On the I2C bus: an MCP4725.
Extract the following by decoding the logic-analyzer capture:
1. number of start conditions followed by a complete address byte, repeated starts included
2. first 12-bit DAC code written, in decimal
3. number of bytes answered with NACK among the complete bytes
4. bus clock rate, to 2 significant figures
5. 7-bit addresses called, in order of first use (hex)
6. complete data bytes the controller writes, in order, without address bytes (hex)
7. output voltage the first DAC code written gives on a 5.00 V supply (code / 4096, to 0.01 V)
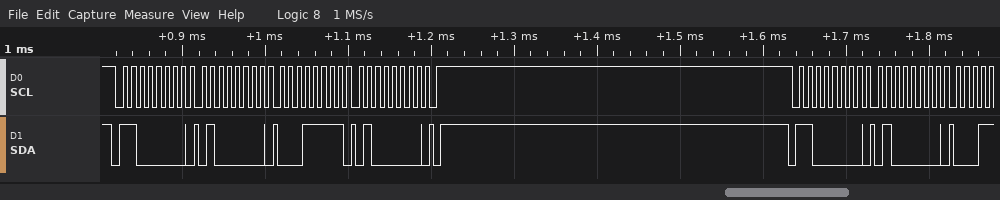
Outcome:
2
500
0
100 kHz
0x60
40 1F 40 40
0.61 V
